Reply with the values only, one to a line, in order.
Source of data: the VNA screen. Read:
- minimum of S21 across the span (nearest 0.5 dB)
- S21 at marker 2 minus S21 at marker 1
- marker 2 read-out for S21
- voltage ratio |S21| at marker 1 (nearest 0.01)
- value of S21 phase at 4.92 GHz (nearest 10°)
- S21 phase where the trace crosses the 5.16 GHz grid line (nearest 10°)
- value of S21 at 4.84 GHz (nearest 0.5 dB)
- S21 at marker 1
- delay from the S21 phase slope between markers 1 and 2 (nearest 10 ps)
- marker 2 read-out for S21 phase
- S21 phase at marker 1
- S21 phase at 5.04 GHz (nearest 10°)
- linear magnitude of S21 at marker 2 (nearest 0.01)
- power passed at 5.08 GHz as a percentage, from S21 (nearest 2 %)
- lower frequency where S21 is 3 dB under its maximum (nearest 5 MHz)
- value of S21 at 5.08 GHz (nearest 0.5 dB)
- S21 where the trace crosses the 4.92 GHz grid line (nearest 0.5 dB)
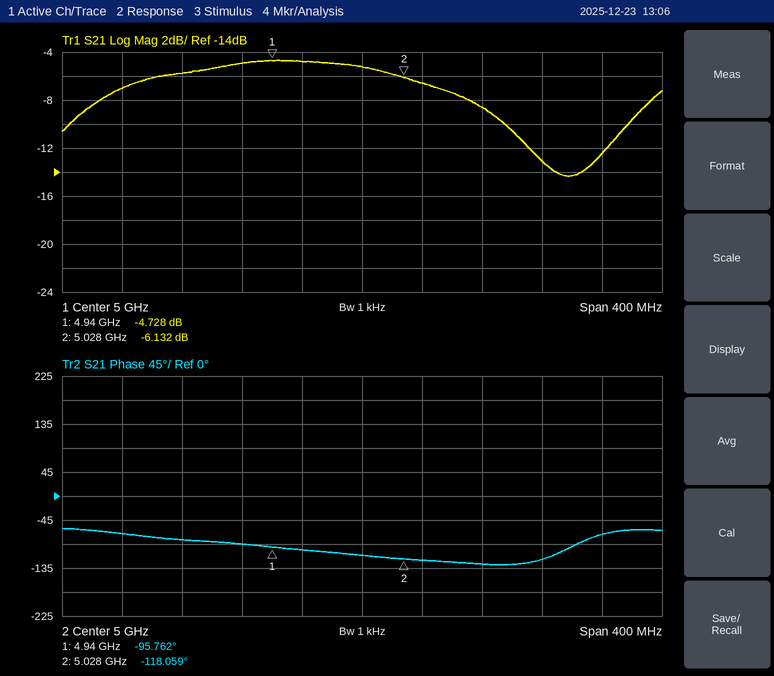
-14.5 dB
-1.404 dB
-6.132 dB
0.58
-90°
-70°
-7.0 dB
-4.728 dB
700 ps
-118.059°
-95.762°
-120°
0.49
14 %
4.830 GHz
-8.5 dB
-5.0 dB
